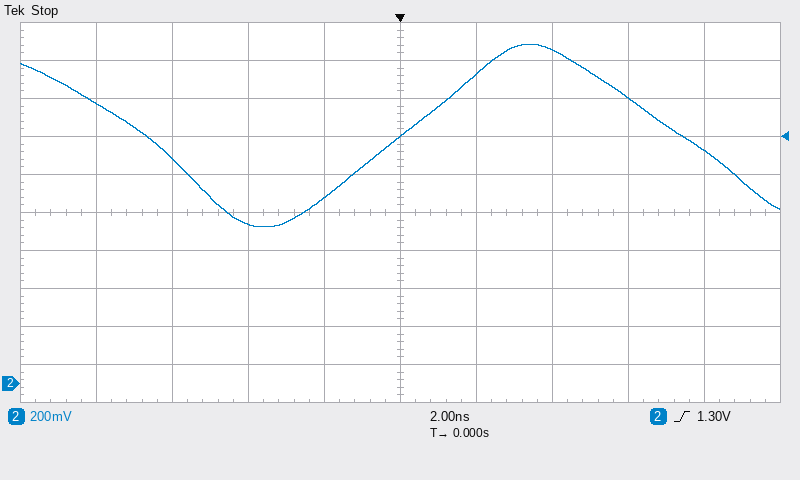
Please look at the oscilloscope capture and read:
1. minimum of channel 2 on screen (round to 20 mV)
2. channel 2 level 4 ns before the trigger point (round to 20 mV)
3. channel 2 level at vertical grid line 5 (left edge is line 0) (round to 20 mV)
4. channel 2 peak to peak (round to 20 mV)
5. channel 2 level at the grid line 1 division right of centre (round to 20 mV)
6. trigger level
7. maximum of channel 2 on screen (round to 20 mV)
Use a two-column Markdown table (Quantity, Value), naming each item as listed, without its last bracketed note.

| Quantity | Value |
|---|---|
| minimum of channel 2 on screen | 820 mV |
| channel 2 level 4 ns before the trigger point | 840 mV |
| channel 2 level at vertical grid line 5 (left edge is line 0) | 1.30 V |
| channel 2 peak to peak | 960 mV |
| channel 2 level at the grid line 1 division right of centre | 1.62 V |
| trigger level | 1.30 V |
| maximum of channel 2 on screen | 1.78 V |
